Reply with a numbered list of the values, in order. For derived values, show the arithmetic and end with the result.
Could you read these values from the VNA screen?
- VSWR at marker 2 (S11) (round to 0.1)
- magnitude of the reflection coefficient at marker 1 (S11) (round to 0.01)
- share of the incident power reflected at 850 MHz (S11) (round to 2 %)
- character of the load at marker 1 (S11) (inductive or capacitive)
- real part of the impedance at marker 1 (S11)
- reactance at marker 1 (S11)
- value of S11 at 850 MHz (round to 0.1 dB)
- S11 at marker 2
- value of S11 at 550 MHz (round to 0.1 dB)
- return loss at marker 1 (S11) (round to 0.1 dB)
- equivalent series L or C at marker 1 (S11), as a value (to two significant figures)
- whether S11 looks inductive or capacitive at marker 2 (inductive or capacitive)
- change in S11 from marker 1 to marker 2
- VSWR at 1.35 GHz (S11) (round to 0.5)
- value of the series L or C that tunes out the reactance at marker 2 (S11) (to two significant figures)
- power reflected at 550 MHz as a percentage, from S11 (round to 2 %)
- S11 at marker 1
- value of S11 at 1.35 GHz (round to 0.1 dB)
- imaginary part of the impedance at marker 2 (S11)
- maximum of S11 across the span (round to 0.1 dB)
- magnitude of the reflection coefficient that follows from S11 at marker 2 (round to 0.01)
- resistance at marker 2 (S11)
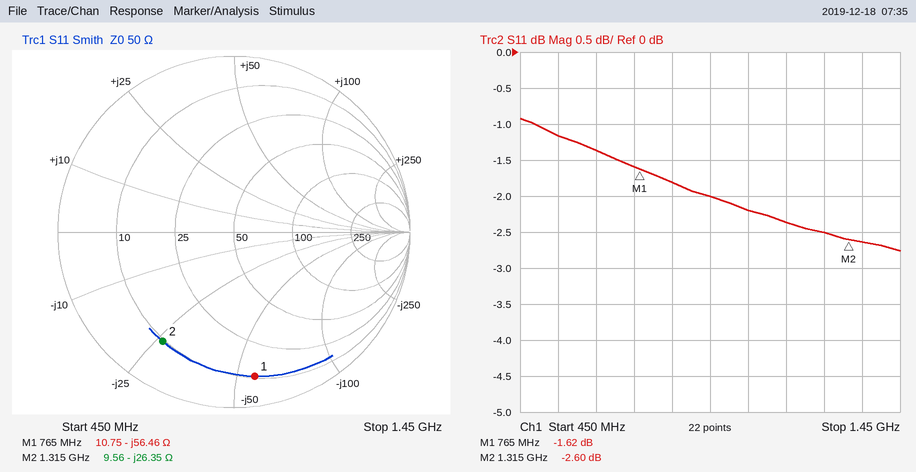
1. 6.7
2. 10^(-1.62/20) ≈ 0.83
3. 10^(-1.8/10) ≈ 66 %
4. capacitive
5. 10.75 Ω
6. -56.46 Ω
7. -1.8 dB
8. -2.60 dB
9. -1.2 dB
10. 1.6 dB
11. C = 1/(2π × 765 MHz × 56.46 Ω) ≈ 3.7 pF
12. capacitive
13. -2.6 − (-1.62) = -0.98 dB
14. |Γ| = 10^(-2.6/20) = 0.7413; VSWR = (1 + 0.7413)/(1 − 0.7413) ≈ 6.73, so 6.5 to the nearest 0.5
15. L = 26.35 Ω/(2π × 1.315 GHz) ≈ 3.2 nH
16. 10^(-1.2/10) ≈ 76 %
17. -1.62 dB
18. -2.6 dB
19. -26.35 Ω
20. -0.9 dB
21. 10^(-2.6/20) ≈ 0.74
22. 9.56 Ω
